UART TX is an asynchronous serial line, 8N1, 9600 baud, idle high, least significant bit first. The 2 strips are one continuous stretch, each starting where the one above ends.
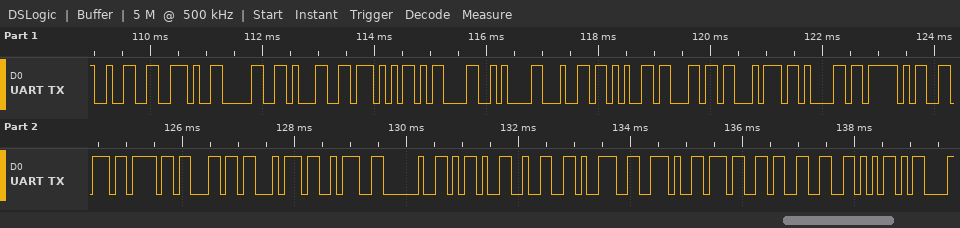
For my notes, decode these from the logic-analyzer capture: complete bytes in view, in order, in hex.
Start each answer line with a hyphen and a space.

- 32 2E 30 31 57 0D 0A 64 65 6C 74 61 5F 76 6F 6C 74 3A 20 2D 32 39 2E 37 33 56 0D
